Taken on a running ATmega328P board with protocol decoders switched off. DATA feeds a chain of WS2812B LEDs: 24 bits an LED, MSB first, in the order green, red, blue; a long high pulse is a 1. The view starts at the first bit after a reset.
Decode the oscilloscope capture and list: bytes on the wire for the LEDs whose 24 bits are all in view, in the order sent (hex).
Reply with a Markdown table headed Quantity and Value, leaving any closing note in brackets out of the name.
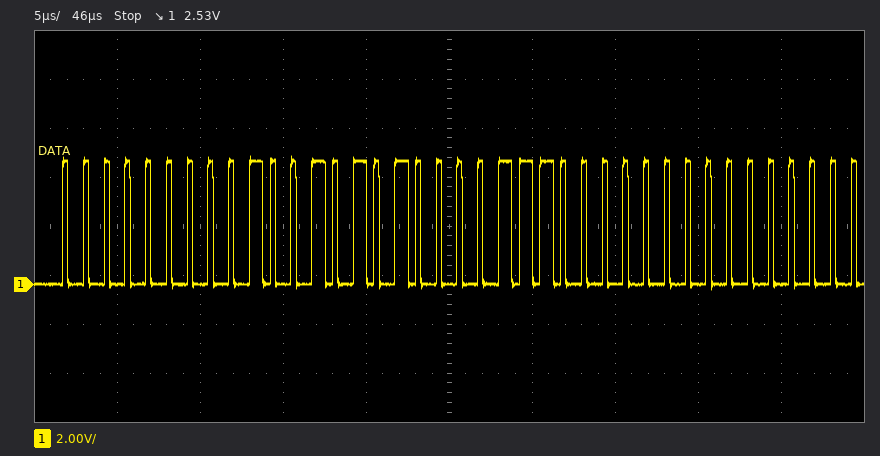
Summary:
| Quantity | Value |
|---|---|
| bytes on the wire for the LEDs whose 24 bits are all in view, in the order sent | 00 4A 87 |
